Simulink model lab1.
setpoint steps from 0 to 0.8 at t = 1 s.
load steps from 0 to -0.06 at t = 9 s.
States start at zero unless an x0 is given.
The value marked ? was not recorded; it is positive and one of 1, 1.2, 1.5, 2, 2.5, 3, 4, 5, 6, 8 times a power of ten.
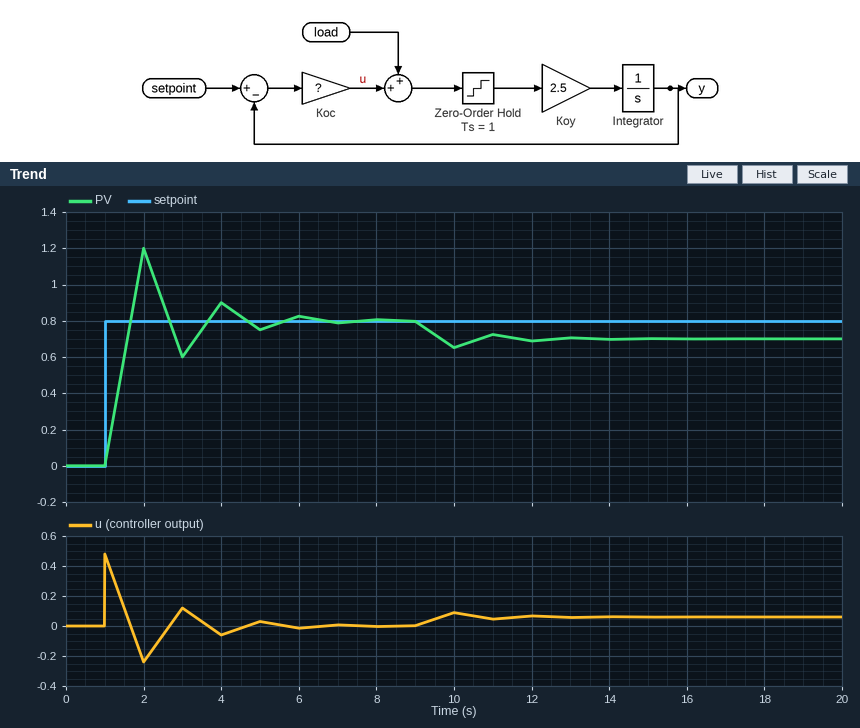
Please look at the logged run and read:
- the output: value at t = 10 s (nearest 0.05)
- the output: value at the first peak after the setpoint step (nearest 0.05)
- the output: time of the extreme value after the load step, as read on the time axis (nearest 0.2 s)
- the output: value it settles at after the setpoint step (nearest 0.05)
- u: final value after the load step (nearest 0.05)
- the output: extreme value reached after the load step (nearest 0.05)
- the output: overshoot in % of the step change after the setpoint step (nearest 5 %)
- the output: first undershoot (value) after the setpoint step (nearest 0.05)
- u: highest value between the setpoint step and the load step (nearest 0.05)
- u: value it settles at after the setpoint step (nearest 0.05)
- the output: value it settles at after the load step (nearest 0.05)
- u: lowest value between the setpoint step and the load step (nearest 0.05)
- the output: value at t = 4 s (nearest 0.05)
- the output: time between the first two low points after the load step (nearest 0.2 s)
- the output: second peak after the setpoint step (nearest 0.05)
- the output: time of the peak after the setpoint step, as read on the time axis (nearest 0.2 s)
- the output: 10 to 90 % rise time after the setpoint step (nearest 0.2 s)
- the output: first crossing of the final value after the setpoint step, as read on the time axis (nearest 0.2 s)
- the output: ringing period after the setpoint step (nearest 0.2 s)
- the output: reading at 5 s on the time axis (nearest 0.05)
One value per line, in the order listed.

0.65
1.20
10.0 s
0.80
0.05
0.65
50 %
0.60
0.50
0.00
0.70
-0.25
0.90
2.0 s
0.90
2.0 s
0.6 s
1.6 s
2.0 s
0.75
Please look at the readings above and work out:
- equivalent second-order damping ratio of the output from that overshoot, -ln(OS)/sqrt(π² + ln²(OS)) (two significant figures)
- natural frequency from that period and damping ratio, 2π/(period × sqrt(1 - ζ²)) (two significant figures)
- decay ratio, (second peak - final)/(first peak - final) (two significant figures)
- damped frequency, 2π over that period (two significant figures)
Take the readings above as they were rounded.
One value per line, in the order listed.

0.22
3.2 rad/s
0.25
3.1 rad/s
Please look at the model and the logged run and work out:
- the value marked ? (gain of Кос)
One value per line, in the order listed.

0.6
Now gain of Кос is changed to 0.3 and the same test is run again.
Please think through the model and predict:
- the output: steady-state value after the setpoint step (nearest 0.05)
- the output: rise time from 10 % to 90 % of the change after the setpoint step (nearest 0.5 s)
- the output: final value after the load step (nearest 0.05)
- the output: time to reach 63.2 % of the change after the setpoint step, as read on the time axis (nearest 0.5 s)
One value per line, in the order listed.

0.80
1.5 s
0.60
2.0 s
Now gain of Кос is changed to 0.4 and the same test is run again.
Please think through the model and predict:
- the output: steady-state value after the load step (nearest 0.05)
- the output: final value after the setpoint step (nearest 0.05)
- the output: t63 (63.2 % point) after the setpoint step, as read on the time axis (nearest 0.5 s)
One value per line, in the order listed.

0.65
0.80
1.5 s
